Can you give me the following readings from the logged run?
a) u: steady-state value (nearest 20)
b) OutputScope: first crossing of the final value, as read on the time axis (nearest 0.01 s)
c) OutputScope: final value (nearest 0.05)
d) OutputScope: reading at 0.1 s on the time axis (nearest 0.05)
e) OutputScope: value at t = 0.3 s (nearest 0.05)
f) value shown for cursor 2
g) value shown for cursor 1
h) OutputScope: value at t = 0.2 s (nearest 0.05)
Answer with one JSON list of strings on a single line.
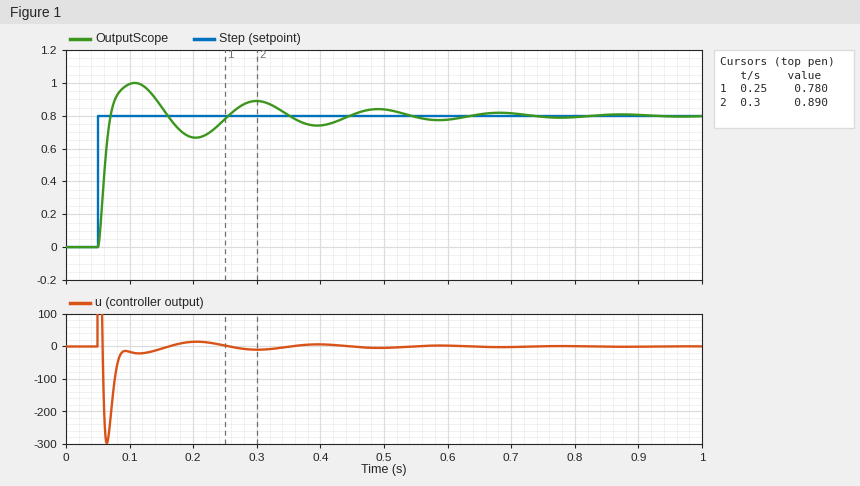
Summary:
["0", "0.07 s", "0.80", "1.00", "0.90", "0.890", "0.780", "0.65"]
